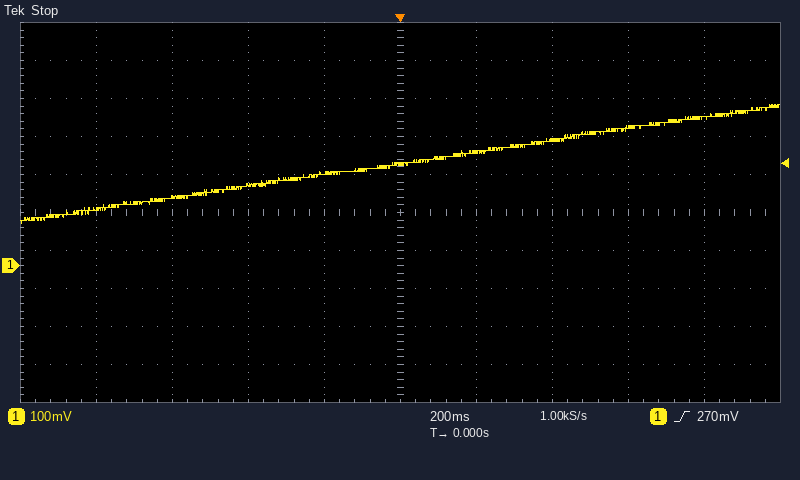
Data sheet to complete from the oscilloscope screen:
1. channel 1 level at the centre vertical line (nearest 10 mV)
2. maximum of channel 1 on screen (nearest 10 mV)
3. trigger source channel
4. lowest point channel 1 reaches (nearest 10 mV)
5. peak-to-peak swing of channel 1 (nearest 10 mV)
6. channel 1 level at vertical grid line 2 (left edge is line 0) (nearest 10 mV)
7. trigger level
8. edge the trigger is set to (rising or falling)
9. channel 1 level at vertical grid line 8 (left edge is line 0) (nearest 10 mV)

270 mV
420 mV
channel 1
110 mV
310 mV
180 mV
270 mV
rising
360 mV
